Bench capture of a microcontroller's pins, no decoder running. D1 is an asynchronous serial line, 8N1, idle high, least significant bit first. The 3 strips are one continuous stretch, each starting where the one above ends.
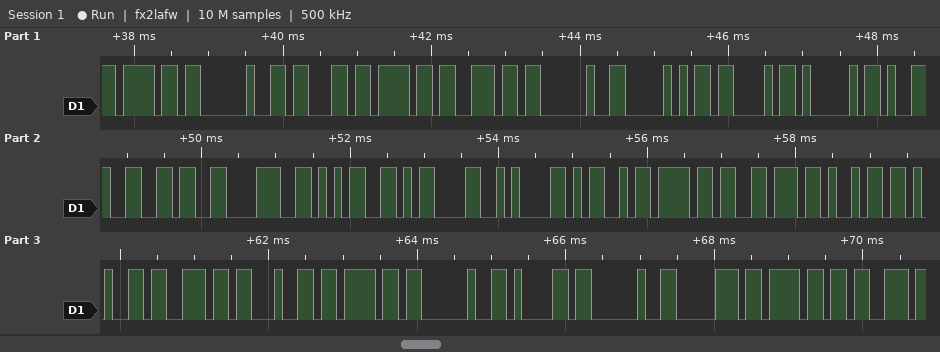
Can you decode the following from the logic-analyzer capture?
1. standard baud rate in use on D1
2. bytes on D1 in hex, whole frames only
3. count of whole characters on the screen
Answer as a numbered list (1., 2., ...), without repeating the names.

1. 9600 baud
2. 6F 20 63 6F 6E 20 50 43 41 39 36 38 35 0D 0A 4D 6F 76 69 65 6E 64 6F 20 61 20 70 6F 73
3. 29
